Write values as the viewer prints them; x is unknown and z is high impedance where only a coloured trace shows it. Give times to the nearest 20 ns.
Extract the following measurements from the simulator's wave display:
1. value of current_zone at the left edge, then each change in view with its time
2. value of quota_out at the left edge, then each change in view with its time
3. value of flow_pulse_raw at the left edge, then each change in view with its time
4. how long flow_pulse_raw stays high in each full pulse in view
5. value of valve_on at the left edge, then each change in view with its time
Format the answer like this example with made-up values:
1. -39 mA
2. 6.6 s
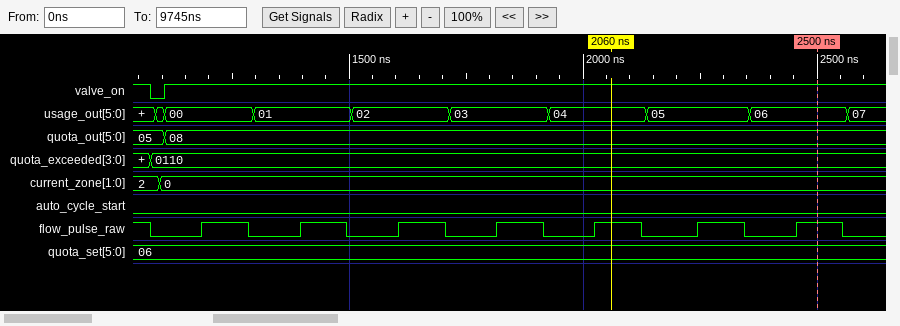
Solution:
1. 2, 0 at 1100 ns
2. 05, 08 at 1100 ns
3. 1, 0 at 1080 ns, 1 at 1180 ns, 0 at 1280 ns, 1 at 1400 ns, 0 at 1500 ns, 1 at 1600 ns, 0 at 1700 ns, 1 at 1820 ns, 0 at 1920 ns, 1 at 2020 ns, 0 at 2120 ns, 1 at 2240 ns, 0 at 2340 ns, 1 at 2460 ns, 0 at 2560 ns
4. 100 ns, 100 ns, 100 ns, 100 ns, 100 ns, 100 ns, 100 ns
5. 1, 0 at 1080 ns, 1 at 1100 ns
